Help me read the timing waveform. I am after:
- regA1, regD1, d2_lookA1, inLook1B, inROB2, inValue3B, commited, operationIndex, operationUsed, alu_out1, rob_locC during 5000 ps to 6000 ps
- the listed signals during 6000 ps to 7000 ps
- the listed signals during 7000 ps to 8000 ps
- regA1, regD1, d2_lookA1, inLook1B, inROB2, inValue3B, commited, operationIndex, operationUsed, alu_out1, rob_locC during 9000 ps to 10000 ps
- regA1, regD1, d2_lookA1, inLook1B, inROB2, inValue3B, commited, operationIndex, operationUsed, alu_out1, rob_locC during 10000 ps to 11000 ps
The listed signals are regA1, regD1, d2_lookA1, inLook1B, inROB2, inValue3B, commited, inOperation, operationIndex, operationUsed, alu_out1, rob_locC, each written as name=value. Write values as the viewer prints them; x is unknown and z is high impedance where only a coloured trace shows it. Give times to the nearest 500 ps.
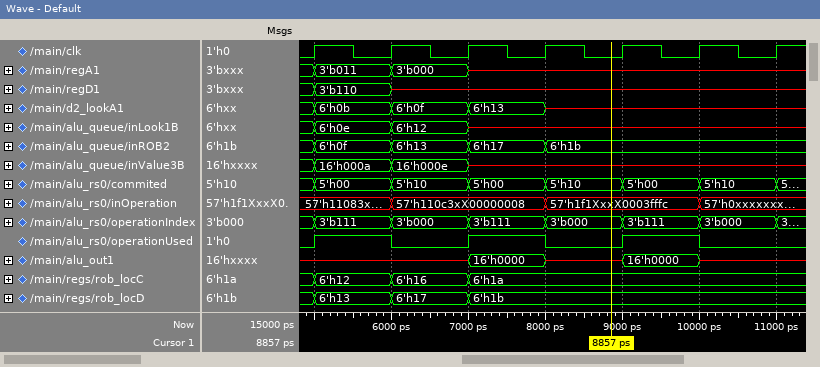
regA1=3'b011, regD1=3'b110, d2_lookA1=6'h0b, inLook1B=6'h0e, inROB2=6'h0f, inValue3B=16'h000a, commited=5'h00, operationIndex=3'b111, operationUsed=1, alu_out1=x, rob_locC=6'h12
regA1=3'b000, regD1=x, d2_lookA1=6'h0f, inLook1B=6'h12, inROB2=6'h13, inValue3B=16'h000e, commited=5'h10, inOperation=57'h110c3xX00000008, operationIndex=3'b000, operationUsed=0, alu_out1=x, rob_locC=6'h16
regA1=x, regD1=x, d2_lookA1=6'h13, inLook1B=x, inROB2=6'h17, inValue3B=x, commited=5'h00, inOperation=57'h110c3xX00000008, operationIndex=3'b111, operationUsed=1, alu_out1=16'h0000, rob_locC=6'h1a
regA1=x, regD1=x, d2_lookA1=x, inLook1B=x, inROB2=6'h1b, inValue3B=x, commited=5'h00, operationIndex=3'b111, operationUsed=1, alu_out1=16'h0000, rob_locC=6'h1a
regA1=x, regD1=x, d2_lookA1=x, inLook1B=x, inROB2=6'h1b, inValue3B=x, commited=5'h10, operationIndex=3'b000, operationUsed=0, alu_out1=x, rob_locC=6'h1a
